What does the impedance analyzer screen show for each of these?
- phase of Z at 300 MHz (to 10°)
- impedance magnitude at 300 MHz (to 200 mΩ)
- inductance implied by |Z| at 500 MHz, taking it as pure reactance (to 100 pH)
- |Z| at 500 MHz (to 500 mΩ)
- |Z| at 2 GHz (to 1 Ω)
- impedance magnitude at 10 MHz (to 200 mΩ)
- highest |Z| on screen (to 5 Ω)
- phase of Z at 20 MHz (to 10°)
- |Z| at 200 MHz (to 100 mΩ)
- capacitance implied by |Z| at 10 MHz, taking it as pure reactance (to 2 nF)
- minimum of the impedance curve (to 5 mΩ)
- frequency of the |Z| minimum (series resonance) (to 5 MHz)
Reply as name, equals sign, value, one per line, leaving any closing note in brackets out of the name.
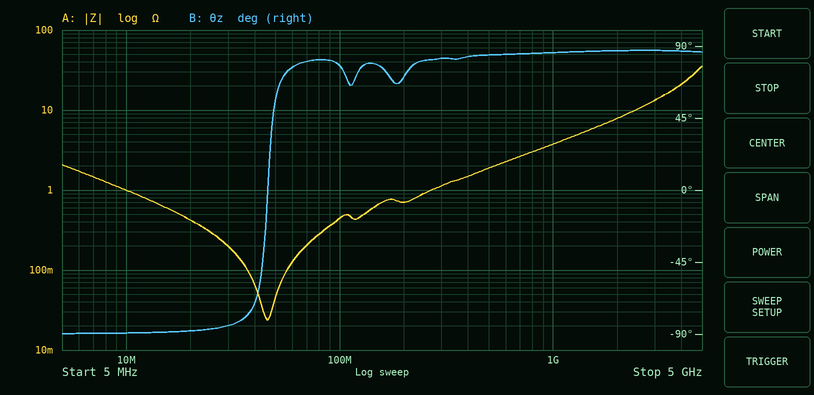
phase of Z at 300 MHz = 80°
impedance magnitude at 300 MHz = 1.2 Ω
inductance implied by |Z| at 500 MHz, taking it as pure reactance = 600 pH
|Z| at 500 MHz = 2.0 Ω
|Z| at 2 GHz = 8 Ω
impedance magnitude at 10 MHz = 1.0 Ω
highest |Z| on screen = 35 Ω
phase of Z at 20 MHz = -90°
|Z| at 200 MHz = 700 mΩ
capacitance implied by |Z| at 10 MHz, taking it as pure reactance = 16 nF
minimum of the impedance curve = 25 mΩ
frequency of the |Z| minimum (series resonance) = 45 MHz
